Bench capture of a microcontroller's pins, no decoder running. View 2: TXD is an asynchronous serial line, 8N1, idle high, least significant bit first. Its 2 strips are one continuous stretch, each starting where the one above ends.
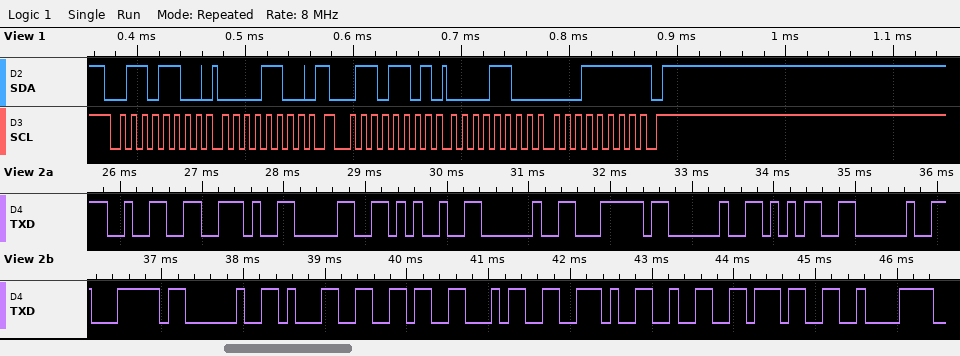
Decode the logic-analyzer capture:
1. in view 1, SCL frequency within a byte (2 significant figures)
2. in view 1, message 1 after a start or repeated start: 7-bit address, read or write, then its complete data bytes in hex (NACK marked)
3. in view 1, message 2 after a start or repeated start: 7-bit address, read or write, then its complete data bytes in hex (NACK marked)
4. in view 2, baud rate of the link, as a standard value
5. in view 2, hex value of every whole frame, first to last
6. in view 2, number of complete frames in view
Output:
100 kHz
0x36 write: 0C
0x36 read: 0C 1F NACK
9600 baud
32 2E 30 25 20 7C 20 35 20 7C 20 31 36 34 2E 32 37 C2
18
